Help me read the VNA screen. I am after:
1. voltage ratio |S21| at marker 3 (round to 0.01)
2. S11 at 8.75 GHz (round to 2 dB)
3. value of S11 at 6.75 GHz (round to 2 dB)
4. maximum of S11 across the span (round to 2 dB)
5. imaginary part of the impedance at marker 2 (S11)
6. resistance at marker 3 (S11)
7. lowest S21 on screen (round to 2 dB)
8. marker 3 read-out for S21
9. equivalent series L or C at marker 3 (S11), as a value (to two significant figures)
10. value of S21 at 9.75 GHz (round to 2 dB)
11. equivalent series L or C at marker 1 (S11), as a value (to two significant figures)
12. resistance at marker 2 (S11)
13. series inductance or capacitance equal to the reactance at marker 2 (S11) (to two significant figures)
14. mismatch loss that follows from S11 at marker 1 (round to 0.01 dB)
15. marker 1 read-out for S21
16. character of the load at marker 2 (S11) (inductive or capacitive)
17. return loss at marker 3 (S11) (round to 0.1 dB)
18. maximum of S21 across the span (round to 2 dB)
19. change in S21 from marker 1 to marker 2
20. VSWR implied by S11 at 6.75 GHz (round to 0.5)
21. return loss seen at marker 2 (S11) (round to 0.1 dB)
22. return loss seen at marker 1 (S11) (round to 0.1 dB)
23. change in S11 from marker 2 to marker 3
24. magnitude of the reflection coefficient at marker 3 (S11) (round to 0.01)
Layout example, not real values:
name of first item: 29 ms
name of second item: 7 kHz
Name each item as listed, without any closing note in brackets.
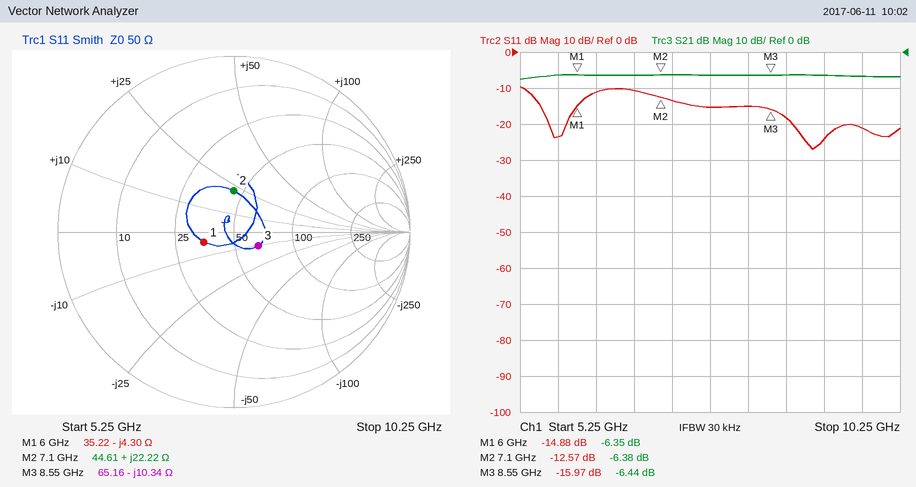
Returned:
voltage ratio |S21| at marker 3: 0.48
S11 at 8.75 GHz: -18 dB
value of S11 at 6.75 GHz: -10 dB
maximum of S11 across the span: -10 dB
imaginary part of the impedance at marker 2: +22.22 Ω
resistance at marker 3: 65.16 Ω
lowest S21 on screen: -8 dB
marker 3 read-out for S21: -6.44 dB
equivalent series L or C at marker 3 (S11), as a value: 1.8 pF
value of S21 at 9.75 GHz: -6 dB
equivalent series L or C at marker 1 (S11), as a value: 6.2 pF
resistance at marker 2: 44.61 Ω
series inductance or capacitance equal to the reactance at marker 2 (S11): 500 pH
mismatch loss that follows from S11 at marker 1: 0.14 dB
marker 1 read-out for S21: -6.35 dB
character of the load at marker 2 (S11): inductive
return loss at marker 3 (S11): 16.0 dB
maximum of S21 across the span: -6 dB
change in S21 from marker 1 to marker 2: -0.03 dB
VSWR implied by S11 at 6.75 GHz: 2.0
return loss seen at marker 2 (S11): 12.6 dB
return loss seen at marker 1 (S11): 14.9 dB
change in S11 from marker 2 to marker 3: -3.40 dB
magnitude of the reflection coefficient at marker 3 (S11): 0.16
